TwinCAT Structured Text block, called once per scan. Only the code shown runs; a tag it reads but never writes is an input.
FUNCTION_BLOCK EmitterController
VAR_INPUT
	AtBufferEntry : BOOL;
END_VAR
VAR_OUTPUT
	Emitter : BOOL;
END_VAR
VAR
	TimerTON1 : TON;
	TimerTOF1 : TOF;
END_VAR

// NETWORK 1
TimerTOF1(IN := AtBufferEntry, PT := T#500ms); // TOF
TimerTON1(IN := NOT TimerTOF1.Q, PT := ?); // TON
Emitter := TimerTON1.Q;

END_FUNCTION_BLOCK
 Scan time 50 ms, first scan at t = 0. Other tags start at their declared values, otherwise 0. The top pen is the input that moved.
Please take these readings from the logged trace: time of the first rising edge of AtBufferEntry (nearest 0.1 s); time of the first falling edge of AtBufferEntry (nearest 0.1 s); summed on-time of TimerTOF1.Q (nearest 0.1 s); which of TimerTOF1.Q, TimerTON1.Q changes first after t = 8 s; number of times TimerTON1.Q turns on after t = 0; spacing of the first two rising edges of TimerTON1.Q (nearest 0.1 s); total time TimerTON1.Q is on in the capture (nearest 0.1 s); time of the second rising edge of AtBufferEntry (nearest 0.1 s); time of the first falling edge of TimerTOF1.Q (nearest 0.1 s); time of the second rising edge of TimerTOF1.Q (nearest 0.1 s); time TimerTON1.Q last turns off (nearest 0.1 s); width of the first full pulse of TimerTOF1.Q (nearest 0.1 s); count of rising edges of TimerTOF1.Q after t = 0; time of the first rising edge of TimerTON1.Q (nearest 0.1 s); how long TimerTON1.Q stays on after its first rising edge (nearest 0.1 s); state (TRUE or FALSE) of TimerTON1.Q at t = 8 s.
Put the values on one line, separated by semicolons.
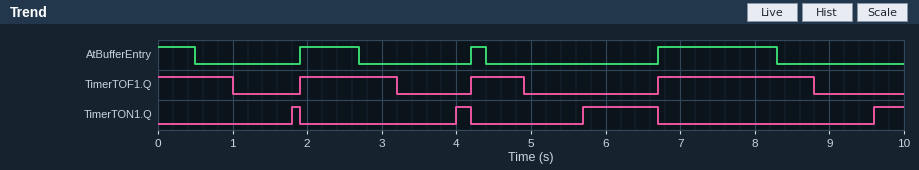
1.9 s; 0.5 s; 5.1 s; TimerTOF1.Q; 4; 2.2 s; 1.7 s; 4.2 s; 1.0 s; 4.2 s; 6.7 s; 1.3 s; 3; 1.8 s; 0.1 s; FALSE
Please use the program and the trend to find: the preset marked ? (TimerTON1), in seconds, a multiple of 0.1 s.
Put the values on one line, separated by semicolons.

0.8 s
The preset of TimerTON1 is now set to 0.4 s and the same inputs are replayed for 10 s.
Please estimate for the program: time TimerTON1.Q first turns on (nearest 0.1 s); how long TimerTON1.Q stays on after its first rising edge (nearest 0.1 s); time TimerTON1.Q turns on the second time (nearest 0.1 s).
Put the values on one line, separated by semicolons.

1.4 s; 0.5 s; 3.6 s
